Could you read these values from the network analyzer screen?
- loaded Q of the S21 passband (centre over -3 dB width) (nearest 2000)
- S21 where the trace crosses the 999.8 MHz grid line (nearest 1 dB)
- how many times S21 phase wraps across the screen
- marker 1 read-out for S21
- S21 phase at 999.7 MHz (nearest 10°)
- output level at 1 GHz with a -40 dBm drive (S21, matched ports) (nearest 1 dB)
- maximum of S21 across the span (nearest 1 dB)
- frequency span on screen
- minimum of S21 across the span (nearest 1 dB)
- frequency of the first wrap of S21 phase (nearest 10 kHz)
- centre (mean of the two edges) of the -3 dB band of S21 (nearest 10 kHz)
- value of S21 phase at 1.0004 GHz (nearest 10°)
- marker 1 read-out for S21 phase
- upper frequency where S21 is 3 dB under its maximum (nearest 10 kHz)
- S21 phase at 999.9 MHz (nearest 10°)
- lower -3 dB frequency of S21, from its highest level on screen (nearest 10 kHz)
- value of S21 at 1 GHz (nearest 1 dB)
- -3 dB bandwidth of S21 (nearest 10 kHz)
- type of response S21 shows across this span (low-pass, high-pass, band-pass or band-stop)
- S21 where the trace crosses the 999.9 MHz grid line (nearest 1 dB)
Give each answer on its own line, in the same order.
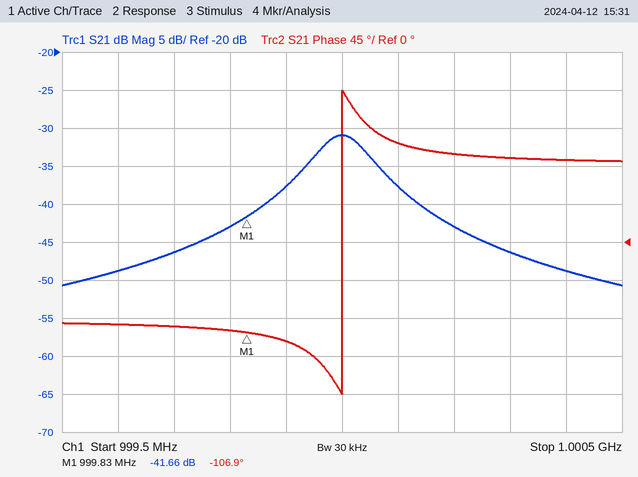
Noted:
10000
-43 dB
1
-41.66 dB
-100°
-71 dBm
-31 dB
1 MHz
-51 dB
1.00000 GHz
1.00000 GHz
100°
-106.9°
1.00005 GHz
-120°
999.95 MHz
-31 dB
100 kHz
band-pass
-38 dB
